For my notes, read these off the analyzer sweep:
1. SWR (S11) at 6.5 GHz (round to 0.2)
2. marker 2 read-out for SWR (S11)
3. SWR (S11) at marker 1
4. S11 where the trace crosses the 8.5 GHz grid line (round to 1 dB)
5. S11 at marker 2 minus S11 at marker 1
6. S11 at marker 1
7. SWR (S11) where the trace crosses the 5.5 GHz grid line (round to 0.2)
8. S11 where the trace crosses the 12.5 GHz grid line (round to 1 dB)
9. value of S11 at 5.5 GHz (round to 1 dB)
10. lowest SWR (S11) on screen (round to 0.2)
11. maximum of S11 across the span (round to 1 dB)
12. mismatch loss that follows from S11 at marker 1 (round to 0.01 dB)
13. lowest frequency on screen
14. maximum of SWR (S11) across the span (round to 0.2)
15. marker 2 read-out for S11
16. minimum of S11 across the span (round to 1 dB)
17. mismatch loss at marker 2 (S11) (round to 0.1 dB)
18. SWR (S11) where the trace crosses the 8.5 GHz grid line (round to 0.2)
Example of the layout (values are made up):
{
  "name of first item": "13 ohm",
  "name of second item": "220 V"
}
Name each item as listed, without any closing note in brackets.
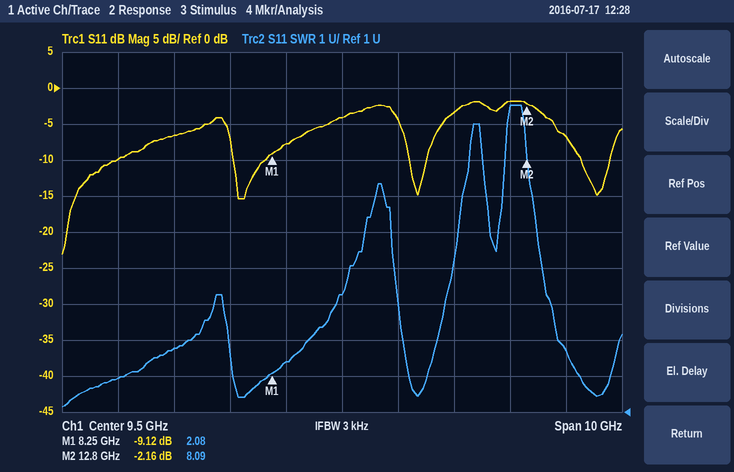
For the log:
{
  "SWR (S11) at 6.5 GHz": "2.8",
  "marker 2 read-out for SWR": "8.09",
  "SWR (S11) at marker 1": "2.08",
  "S11 where the trace crosses the 8.5 GHz grid line": "-8 dB",
  "S11 at marker 2 minus S11 at marker 1": "6.96 dB",
  "S11 at marker 1": "-9.12 dB",
  "SWR (S11) where the trace crosses the 5.5 GHz grid line": "2.0",
  "S11 where the trace crosses the 12.5 GHz grid line": "-2 dB",
  "value of S11 at 5.5 GHz": "-10 dB",
  "lowest SWR (S11) on screen": "1.2",
  "maximum of S11 across the span": "-2 dB",
  "mismatch loss that follows from S11 at marker 1": "0.57 dB",
  "lowest frequency on screen": "4.5 GHz",
  "maximum of SWR (S11) across the span": "9.6",
  "marker 2 read-out for S11": "-2.16 dB",
  "minimum of S11 across the span": "-23 dB",
  "mismatch loss at marker 2 (S11)": "4.1 dB",
  "SWR (S11) where the trace crosses the 8.5 GHz grid line": "2.4"
}
